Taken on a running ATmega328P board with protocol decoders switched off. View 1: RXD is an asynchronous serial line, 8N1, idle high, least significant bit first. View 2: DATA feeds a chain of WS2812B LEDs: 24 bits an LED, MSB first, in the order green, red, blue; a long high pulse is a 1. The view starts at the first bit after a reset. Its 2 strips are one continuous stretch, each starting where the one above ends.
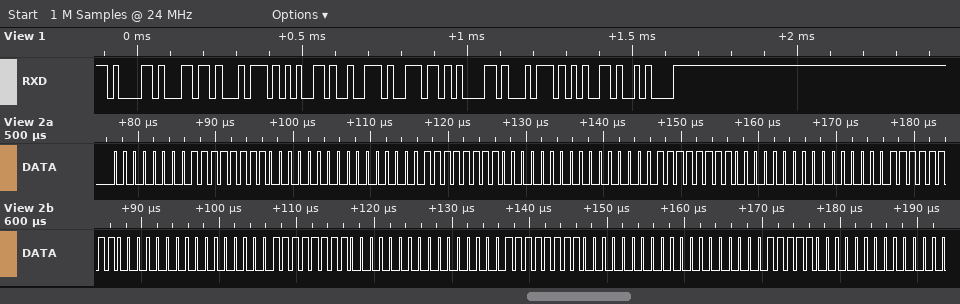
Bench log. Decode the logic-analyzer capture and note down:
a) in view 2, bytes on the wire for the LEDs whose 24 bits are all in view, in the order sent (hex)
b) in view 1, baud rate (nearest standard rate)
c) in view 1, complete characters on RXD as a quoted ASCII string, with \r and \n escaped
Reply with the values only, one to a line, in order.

00 FF 00 00 FF 00 00 FF 00 00 FF 00 00 FF 00 00 FF 00 00 1F 00
57600 baud
"alternate\n"
